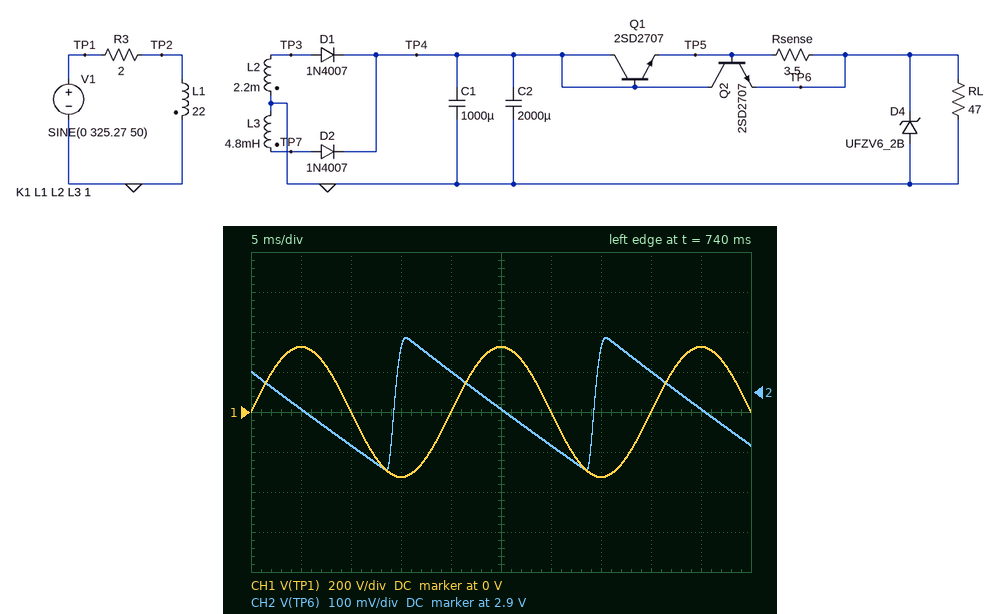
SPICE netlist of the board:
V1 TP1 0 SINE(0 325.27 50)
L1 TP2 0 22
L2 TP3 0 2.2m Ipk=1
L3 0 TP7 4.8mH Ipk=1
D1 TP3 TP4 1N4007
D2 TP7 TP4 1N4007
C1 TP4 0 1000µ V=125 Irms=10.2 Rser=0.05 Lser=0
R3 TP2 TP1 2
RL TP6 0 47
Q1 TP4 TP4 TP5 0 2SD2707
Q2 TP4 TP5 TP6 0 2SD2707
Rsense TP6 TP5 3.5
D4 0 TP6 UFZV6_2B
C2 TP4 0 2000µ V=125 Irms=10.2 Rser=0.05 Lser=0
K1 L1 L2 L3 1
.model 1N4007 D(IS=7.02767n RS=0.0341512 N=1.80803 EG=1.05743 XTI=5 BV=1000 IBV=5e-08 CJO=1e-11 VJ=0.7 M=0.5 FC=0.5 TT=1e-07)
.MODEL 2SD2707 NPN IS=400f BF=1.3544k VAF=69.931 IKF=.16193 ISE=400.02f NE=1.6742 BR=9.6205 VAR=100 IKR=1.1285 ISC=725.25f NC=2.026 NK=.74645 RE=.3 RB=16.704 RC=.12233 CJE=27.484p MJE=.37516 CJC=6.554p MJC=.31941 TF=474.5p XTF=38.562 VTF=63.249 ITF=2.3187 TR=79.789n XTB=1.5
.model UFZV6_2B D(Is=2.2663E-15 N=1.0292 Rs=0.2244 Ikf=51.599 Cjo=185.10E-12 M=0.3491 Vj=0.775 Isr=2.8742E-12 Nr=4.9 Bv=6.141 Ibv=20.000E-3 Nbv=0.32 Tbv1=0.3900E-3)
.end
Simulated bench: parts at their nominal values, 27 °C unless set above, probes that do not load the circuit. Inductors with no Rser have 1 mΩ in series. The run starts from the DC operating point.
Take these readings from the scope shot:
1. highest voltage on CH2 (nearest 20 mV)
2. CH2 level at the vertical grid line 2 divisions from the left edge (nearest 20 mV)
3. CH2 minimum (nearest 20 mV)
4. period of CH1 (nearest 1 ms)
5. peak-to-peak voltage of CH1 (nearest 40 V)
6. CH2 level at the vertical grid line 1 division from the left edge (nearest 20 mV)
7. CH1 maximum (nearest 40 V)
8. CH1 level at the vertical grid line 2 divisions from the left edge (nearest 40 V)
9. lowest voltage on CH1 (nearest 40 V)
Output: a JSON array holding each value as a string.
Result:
["3.04 V", "2.76 V", "2.70 V", "20 ms", "640 V", "2.86 V", "320 V", "0 V", "-320 V"]
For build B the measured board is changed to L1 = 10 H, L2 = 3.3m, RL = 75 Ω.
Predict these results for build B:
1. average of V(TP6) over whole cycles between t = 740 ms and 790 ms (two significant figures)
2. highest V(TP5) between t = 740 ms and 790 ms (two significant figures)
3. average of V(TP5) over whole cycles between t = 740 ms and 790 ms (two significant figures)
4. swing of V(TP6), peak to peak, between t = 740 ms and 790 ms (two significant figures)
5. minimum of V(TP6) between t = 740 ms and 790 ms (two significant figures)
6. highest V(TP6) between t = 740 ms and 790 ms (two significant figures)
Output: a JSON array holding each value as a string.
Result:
["5.1 V", "5.6 V", "5.4 V", "390 mV", "4.9 V", "5.3 V"]
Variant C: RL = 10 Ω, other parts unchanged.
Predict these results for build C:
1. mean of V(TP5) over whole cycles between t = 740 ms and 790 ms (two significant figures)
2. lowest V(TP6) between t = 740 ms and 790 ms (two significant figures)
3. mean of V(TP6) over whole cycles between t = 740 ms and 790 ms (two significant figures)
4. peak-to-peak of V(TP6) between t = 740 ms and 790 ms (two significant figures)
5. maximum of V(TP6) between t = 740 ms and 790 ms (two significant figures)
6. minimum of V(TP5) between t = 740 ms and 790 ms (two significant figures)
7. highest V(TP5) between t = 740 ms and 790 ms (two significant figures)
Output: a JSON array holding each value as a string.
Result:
["2.6 V", "1.5 V", "1.9 V", "890 mV", "2.4 V", "2.1 V", "3.1 V"]
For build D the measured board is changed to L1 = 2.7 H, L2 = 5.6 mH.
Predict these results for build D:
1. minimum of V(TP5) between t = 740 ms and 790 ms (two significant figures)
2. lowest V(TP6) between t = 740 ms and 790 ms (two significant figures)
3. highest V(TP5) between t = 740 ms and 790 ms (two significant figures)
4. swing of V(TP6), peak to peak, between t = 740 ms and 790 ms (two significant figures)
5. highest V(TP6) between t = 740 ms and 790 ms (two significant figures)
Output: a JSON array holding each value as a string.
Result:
["8.1 V", "6.4 V", "9.5 V", "140 mV", "6.5 V"]
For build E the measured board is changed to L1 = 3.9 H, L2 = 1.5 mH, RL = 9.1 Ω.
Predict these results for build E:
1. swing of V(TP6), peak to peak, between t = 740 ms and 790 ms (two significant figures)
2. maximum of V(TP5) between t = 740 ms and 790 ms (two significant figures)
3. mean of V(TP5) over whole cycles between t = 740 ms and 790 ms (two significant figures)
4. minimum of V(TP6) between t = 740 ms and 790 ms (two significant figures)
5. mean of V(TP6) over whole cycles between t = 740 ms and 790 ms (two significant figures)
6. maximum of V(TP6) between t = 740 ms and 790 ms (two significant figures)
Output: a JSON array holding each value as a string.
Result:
["1.7 V", "8.3 V", "7.0 V", "4.6 V", "5.7 V", "6.3 V"]
